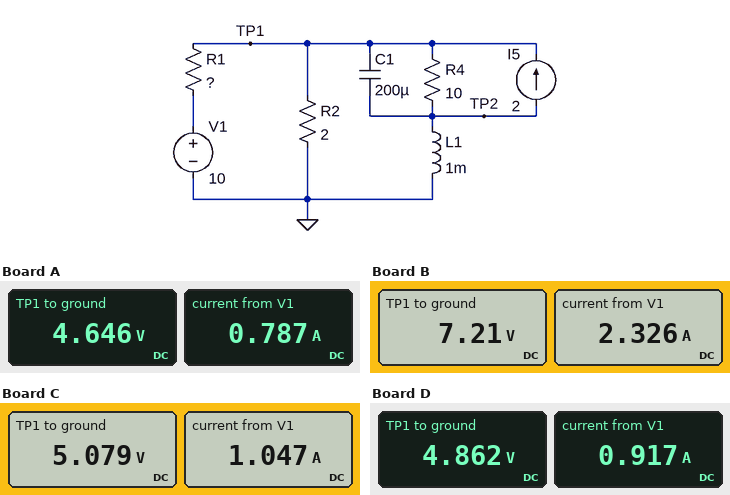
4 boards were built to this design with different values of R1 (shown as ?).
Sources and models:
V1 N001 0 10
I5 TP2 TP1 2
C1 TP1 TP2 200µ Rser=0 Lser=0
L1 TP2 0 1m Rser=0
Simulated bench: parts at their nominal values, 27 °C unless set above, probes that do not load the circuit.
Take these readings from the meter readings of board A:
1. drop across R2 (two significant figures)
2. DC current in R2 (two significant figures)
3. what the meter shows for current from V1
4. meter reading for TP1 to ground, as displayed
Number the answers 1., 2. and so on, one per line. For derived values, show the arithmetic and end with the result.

1. 4.646 V = 4.6 V
2. (4.646 V) / 2 Ω = 2.3 A
3. 0.787 A
4. 4.646 V
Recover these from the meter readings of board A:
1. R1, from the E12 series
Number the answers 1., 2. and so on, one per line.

1. 6.8 Ω
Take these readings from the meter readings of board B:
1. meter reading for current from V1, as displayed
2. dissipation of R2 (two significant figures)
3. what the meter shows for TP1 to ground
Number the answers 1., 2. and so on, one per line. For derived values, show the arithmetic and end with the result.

1. 2.326 A
2. (7.21 V)^2 / 2 Ω = 26 W
3. 7.21 V
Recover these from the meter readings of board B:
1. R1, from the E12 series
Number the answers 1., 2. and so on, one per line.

1. 1.2 Ω
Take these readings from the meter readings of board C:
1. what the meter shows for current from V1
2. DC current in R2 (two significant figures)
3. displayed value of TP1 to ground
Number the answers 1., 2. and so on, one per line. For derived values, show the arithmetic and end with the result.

1. 1.047 A
2. (5.079 V) / 2 Ω = 2.5 A
3. 5.079 V
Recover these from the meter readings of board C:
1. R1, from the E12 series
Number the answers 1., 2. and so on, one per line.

1. 4.7 Ω
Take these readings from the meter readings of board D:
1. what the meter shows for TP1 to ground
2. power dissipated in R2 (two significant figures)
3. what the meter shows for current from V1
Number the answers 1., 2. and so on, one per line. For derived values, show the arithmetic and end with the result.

1. 4.862 V
2. (4.862 V)^2 / 2 Ω = 12 W
3. 0.917 A
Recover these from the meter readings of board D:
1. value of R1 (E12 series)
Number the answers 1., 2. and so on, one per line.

1. 5.6 Ω
